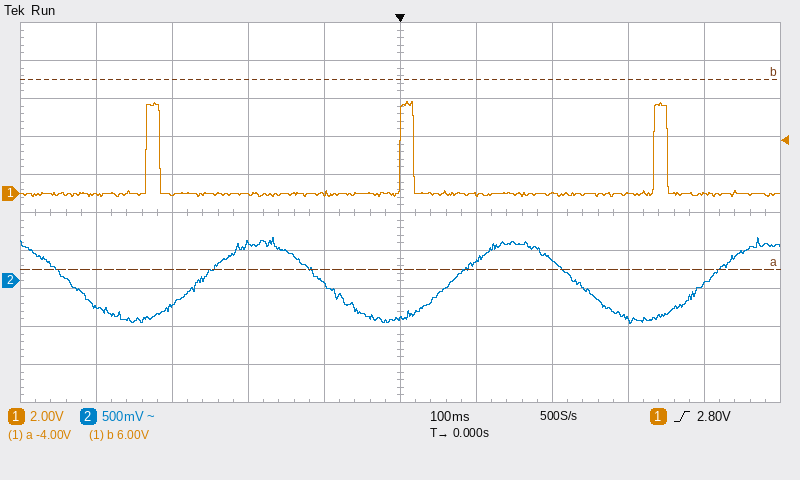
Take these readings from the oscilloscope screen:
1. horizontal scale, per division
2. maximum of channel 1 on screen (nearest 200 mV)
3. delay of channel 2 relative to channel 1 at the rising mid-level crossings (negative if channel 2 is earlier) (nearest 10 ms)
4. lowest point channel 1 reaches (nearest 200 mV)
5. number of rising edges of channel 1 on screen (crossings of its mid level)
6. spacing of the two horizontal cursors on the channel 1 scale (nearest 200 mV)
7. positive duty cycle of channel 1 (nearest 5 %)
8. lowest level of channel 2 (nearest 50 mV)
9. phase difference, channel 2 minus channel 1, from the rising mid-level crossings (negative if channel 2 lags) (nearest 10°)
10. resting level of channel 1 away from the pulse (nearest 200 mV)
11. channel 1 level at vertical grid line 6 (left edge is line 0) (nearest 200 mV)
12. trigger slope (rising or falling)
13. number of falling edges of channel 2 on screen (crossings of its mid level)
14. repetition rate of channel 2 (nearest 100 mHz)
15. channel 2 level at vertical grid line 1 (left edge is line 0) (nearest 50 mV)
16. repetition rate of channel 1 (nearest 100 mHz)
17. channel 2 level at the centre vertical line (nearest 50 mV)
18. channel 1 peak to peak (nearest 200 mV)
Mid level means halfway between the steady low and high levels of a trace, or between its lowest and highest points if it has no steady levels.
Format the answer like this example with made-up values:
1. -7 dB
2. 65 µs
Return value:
1. 100 ms
2. 4.8 V
3. +70 ms
4. -200 mV
5. 3
6. 10.0 V
7. 5 %
8. -550 mV
9. -80°
10. 0.0 V
11. 0.0 V
12. rising
13. 3
14. 3.0 Hz
15. -350 mV
16. 3.0 Hz
17. -500 mV
18. 5.0 V
